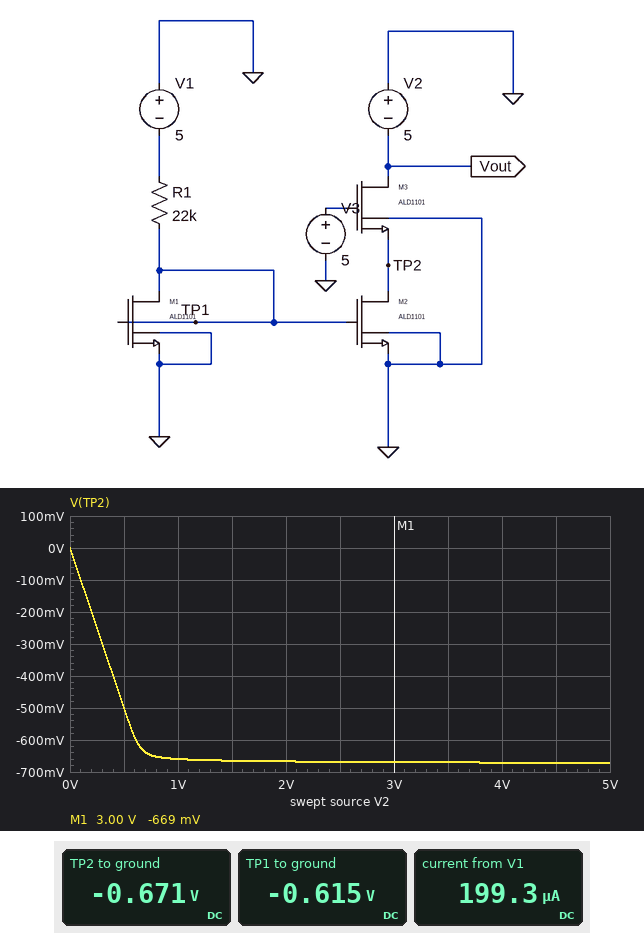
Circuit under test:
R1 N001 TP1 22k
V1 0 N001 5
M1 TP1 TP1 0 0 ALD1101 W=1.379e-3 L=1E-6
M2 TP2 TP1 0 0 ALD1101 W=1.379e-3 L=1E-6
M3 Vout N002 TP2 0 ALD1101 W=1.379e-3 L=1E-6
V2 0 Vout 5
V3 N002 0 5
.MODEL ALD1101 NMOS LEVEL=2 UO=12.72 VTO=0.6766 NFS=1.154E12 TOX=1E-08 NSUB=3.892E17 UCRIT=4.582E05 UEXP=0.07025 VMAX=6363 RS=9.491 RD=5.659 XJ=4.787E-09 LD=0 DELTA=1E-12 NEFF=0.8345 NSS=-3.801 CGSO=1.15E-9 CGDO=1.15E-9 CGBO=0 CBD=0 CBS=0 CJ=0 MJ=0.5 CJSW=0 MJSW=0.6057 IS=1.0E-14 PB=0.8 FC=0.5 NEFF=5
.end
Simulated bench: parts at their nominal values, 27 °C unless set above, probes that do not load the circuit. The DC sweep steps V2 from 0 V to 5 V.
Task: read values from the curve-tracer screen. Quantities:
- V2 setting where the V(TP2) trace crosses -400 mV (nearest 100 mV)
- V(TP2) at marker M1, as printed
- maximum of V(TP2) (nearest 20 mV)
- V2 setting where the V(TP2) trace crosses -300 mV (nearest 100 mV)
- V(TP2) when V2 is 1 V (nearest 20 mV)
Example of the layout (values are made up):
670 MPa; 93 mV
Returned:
400 mV; -669 mV; 0 V; 300 mV; -660 mV
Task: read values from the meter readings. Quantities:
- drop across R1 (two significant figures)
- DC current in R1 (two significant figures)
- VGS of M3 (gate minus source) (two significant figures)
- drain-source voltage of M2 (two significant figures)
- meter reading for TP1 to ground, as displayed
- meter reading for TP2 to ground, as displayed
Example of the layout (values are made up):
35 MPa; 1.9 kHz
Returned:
4.4 V; 200 µA; 5.7 V; -670 mV; -0.615 V; -0.671 V
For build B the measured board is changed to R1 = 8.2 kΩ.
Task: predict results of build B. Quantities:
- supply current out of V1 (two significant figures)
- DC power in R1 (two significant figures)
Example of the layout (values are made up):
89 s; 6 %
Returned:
530 µA; 2.3 mW
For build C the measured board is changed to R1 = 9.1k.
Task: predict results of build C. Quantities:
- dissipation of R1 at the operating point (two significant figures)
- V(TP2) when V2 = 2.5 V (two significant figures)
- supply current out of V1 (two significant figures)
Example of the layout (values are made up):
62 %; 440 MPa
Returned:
2.1 mW; -670 mV; 480 µA
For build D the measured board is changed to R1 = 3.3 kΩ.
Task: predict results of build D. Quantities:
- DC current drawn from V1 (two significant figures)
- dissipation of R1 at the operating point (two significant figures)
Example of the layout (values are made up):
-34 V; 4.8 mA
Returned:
1.3 mA; 5.7 mW
